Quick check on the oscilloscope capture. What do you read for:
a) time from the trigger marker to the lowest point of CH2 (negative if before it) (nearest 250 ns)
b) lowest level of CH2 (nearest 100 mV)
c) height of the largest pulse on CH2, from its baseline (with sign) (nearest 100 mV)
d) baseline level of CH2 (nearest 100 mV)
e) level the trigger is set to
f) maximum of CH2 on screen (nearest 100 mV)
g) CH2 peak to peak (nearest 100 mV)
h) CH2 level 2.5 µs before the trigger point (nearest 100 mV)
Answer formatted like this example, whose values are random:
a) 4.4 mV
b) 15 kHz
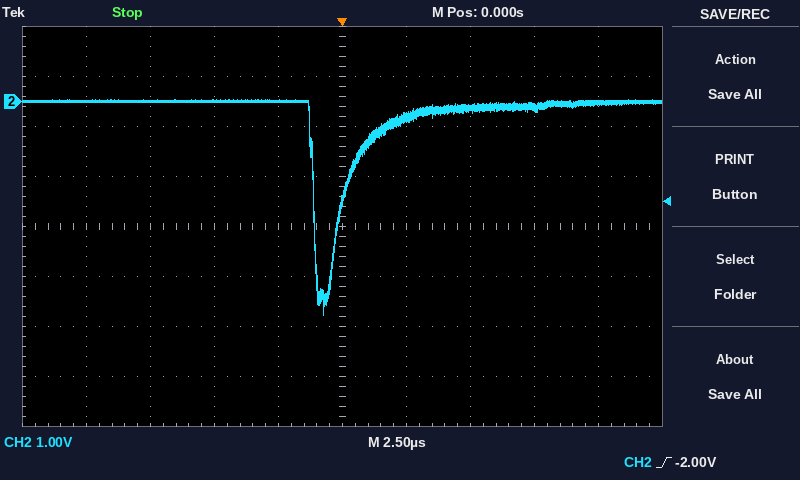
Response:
a) -750 ns
b) -4.3 V
c) -4.3 V
d) 0.0 V
e) -2.00 V
f) 0.0 V
g) 4.3 V
h) 0.0 V
